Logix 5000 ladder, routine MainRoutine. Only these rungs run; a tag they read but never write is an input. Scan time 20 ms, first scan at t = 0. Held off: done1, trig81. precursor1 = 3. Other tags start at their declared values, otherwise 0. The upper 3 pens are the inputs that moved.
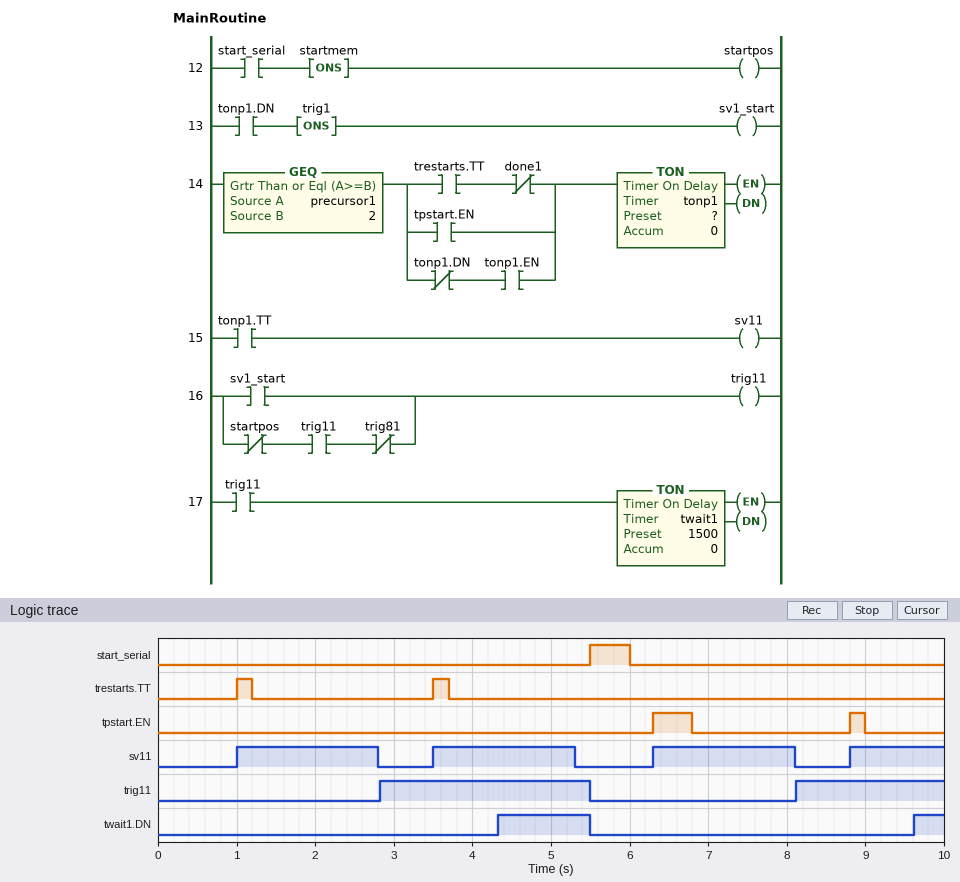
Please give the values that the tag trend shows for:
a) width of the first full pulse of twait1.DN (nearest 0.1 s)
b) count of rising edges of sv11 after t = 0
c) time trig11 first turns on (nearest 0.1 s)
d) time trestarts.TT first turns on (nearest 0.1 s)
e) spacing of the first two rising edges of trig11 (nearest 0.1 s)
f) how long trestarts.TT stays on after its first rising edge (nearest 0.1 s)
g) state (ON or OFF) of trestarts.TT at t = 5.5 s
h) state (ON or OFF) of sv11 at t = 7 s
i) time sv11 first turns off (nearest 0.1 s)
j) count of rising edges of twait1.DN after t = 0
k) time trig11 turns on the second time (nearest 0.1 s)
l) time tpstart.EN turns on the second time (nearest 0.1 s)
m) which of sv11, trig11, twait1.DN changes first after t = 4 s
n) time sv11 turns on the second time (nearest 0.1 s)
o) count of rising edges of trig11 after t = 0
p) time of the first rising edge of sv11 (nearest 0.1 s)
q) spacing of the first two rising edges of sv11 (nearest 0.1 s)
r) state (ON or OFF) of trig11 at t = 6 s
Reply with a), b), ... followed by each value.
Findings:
a) 1.2 s
b) 4
c) 2.8 s
d) 1.0 s
e) 5.3 s
f) 0.2 s
g) OFF
h) ON
i) 2.8 s
j) 2
k) 8.1 s
l) 8.8 s
m) twait1.DN
n) 3.5 s
o) 2
p) 1.0 s
q) 2.5 s
r) OFF
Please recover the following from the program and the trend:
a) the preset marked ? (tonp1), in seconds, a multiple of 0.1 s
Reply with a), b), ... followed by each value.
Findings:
a) 1.8 s
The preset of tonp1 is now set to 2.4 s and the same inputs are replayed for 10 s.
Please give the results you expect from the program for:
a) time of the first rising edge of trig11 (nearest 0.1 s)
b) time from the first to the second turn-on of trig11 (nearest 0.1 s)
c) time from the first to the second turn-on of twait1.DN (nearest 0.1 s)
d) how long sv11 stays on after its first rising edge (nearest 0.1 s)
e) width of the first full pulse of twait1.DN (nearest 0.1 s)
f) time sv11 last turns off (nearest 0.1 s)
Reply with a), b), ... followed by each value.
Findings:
a) 3.4 s
b) 2.5 s
c) 2.5 s
d) 2.4 s
e) 0.6 s
f) 8.7 s
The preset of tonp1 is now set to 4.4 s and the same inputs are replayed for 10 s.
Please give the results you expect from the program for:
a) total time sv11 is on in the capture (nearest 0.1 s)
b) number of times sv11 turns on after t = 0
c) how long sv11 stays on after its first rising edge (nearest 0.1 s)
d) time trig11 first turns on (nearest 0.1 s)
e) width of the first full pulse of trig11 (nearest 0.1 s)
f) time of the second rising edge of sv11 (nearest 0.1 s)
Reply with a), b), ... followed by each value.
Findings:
a) 8.1 s
b) 2
c) 4.4 s
d) 5.4 s
e) 0.1 s
f) 6.3 s
